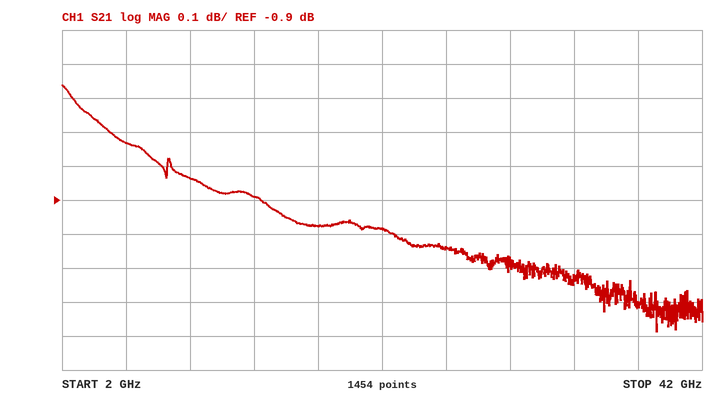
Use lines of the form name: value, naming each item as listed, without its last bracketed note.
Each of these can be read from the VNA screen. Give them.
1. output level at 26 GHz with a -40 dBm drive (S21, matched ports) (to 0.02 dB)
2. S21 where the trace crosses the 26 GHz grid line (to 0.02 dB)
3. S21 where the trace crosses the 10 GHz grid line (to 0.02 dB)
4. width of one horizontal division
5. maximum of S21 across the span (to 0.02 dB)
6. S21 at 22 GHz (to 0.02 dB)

output level at 26 GHz with a -40 dBm drive (S21, matched ports): -41.04 dBm
S21 where the trace crosses the 26 GHz grid line: -1.04 dB
S21 where the trace crosses the 10 GHz grid line: -0.84 dB
width of one horizontal division: 4 GHz
maximum of S21 across the span: -0.56 dB
S21 at 22 GHz: -0.98 dB
